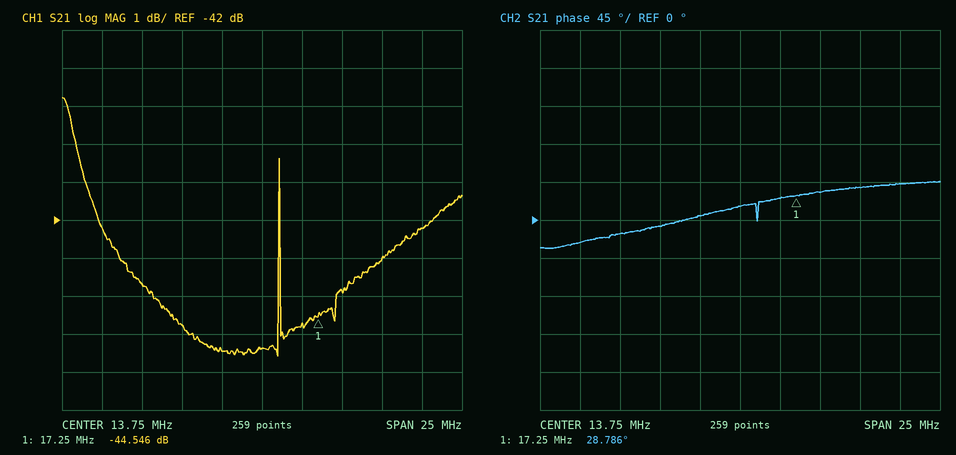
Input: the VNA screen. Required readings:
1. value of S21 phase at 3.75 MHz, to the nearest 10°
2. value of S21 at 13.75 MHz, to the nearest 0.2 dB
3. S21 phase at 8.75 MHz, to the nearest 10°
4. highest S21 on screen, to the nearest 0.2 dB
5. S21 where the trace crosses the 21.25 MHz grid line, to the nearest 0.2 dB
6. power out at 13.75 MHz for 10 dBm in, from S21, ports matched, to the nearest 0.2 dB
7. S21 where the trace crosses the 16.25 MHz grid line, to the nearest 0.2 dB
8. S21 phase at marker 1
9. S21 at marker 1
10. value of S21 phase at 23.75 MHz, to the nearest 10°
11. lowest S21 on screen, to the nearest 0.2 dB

-30°
-45.4 dB
-10°
-38.8 dB
-43.0 dB
-35.4 dBm
-44.8 dB
28.786°
-44.546 dB
40°
-45.6 dB
